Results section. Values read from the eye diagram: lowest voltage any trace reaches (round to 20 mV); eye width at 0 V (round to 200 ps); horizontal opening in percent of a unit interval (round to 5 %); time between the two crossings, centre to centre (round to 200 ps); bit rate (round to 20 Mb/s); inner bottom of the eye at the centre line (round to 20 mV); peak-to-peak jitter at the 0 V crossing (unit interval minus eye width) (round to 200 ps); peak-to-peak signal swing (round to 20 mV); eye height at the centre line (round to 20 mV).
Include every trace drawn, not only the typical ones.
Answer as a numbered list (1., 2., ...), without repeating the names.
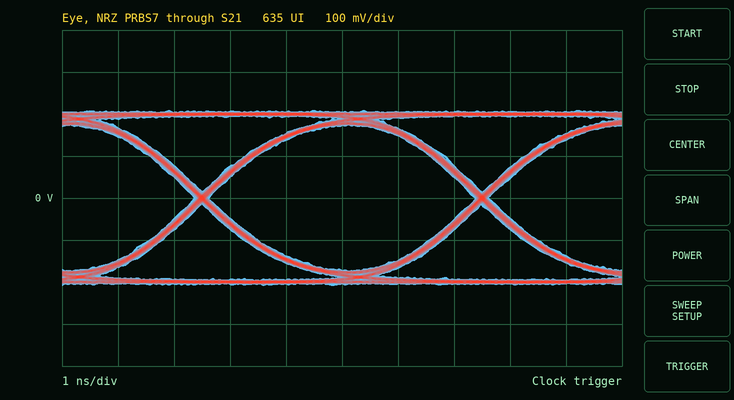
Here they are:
1. -200 mV
2. 4.8 ns
3. 95 %
4. 5.0 ns
5. 200 Mb/s
6. -180 mV
7. 200 ps
8. 420 mV
9. 340 mV
